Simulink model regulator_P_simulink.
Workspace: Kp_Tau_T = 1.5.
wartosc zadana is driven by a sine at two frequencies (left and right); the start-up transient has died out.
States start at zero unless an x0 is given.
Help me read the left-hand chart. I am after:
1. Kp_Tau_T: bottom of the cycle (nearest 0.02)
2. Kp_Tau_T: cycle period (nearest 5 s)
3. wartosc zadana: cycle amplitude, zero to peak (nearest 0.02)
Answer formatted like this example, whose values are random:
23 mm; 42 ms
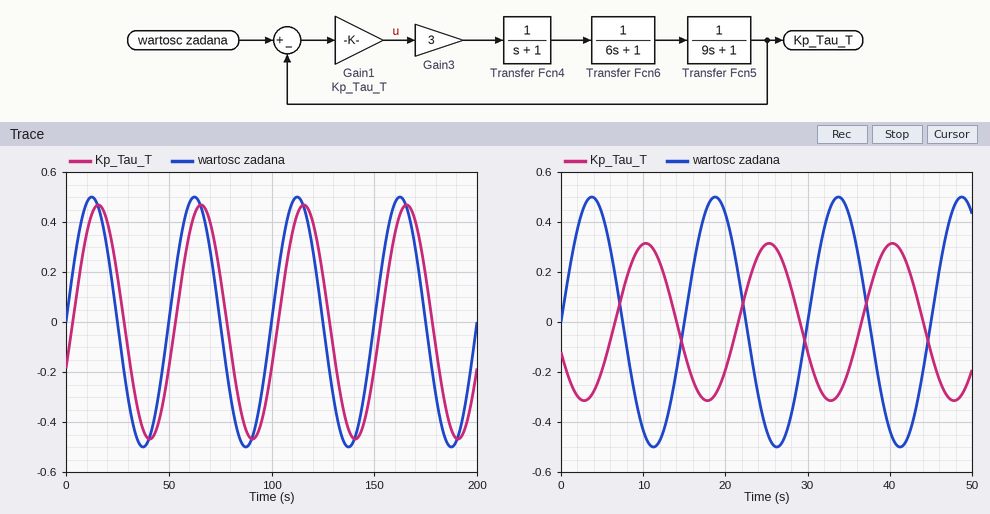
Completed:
-0.46; 50 s; 0.50
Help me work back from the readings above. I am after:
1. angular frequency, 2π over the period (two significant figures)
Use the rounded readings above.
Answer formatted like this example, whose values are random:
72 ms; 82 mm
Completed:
0.13 rad/s
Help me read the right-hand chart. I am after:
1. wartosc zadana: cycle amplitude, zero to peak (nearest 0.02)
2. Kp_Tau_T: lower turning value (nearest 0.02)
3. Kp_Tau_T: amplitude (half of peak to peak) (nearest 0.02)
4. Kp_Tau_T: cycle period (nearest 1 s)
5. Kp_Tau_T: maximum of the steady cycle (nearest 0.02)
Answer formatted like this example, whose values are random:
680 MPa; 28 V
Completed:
0.50; -0.32; 0.32; 15 s; 0.32
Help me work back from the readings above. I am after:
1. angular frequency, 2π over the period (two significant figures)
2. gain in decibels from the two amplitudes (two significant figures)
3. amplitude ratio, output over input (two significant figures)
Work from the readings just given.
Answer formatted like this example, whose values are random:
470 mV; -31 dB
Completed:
0.42 rad/s; -3.9 dB; 0.64
